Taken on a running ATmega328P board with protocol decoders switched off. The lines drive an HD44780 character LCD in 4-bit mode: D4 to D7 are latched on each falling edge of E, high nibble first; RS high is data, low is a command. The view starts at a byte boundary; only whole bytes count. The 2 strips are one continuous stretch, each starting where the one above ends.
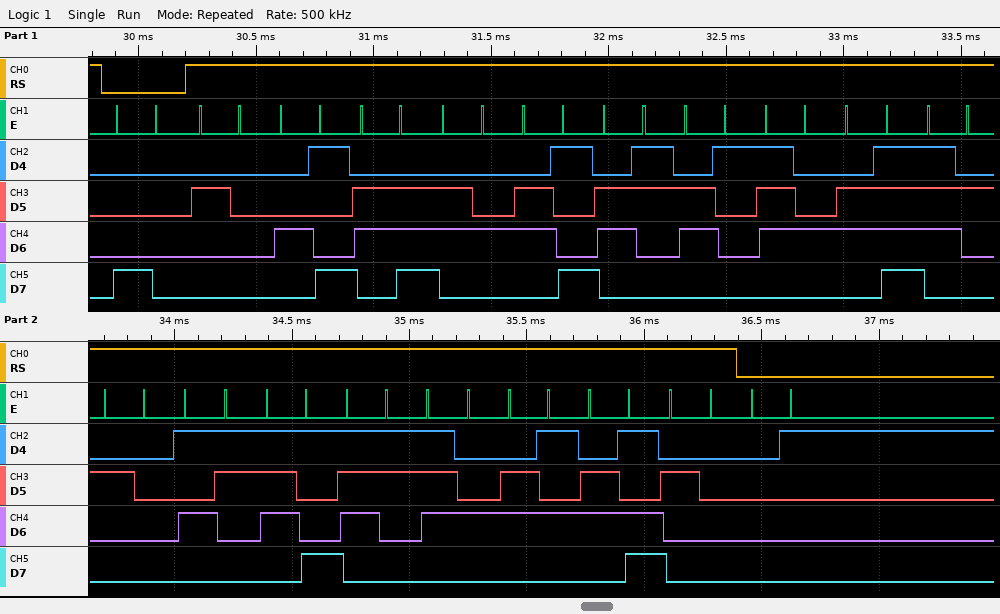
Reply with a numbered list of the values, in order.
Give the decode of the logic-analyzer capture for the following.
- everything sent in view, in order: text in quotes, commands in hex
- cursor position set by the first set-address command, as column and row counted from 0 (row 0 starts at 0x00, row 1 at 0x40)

1. 0x80 " Indicator System " 0x01
2. column 0, row 0
